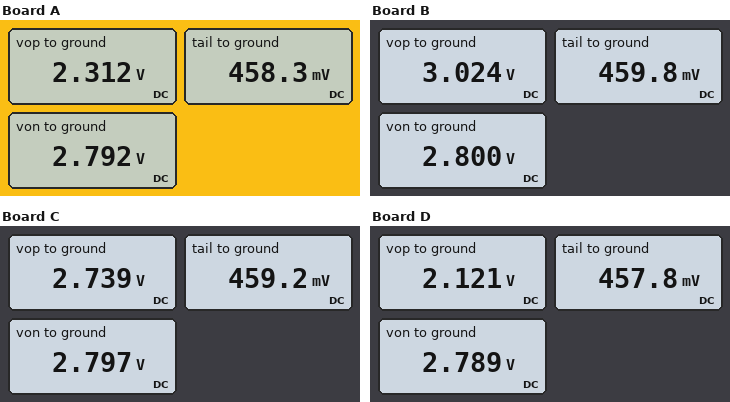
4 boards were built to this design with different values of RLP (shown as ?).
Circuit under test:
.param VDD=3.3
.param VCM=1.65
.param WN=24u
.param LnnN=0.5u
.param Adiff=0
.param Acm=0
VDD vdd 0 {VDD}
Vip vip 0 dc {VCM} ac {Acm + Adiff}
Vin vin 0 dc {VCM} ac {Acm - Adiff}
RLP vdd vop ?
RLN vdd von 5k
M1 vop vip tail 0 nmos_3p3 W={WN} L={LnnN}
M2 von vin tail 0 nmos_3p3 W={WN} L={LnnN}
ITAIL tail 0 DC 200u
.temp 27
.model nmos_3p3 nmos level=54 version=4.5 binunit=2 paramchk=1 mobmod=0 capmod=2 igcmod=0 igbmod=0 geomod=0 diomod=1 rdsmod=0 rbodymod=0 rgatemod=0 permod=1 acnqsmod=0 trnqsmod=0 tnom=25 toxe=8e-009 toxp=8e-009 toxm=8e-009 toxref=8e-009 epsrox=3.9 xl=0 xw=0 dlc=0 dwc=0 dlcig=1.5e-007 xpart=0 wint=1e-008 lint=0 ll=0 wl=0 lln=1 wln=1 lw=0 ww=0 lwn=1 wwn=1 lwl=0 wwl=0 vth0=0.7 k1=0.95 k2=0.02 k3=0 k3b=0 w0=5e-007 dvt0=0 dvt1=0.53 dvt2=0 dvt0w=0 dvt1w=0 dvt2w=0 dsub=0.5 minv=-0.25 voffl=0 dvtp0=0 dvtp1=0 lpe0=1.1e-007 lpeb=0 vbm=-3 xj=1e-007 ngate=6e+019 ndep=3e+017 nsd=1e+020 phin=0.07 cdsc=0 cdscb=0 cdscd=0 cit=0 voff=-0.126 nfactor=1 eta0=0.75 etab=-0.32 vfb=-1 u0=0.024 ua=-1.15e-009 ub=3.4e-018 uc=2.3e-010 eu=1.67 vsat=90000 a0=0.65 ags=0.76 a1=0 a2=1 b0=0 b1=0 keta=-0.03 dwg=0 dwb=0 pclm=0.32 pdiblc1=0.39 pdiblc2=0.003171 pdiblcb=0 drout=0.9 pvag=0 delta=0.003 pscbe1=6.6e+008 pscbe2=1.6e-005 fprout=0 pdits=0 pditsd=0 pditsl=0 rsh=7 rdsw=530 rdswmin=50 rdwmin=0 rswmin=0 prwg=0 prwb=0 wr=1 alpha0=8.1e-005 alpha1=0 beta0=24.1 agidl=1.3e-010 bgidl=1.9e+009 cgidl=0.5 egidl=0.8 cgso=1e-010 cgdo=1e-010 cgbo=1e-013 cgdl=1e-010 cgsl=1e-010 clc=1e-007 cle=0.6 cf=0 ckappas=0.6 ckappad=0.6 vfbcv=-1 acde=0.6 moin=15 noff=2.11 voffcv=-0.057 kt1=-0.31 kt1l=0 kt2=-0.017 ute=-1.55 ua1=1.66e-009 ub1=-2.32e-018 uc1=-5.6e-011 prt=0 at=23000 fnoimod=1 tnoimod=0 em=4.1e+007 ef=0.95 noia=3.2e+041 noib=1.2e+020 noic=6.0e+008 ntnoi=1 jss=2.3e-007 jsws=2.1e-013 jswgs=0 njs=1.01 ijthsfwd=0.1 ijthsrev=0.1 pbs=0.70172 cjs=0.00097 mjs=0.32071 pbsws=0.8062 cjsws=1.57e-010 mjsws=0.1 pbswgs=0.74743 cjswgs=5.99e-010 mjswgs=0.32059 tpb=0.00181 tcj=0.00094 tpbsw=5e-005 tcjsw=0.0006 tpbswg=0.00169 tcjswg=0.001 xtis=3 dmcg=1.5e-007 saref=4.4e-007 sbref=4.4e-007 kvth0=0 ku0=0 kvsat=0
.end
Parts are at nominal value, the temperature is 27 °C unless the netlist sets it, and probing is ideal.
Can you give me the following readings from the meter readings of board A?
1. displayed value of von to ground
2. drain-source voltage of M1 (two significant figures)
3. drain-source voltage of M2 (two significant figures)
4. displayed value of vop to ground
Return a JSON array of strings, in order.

["2.792 V", "1.9 V", "2.3 V", "2.312 V"]
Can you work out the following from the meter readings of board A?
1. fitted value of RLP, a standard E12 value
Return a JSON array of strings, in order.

["10 kΩ"]
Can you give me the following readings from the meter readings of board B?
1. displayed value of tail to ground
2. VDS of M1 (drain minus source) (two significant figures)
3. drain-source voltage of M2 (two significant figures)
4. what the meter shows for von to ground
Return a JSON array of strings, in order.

["459.8 mV", "2.6 V", "2.3 V", "2.800 V"]
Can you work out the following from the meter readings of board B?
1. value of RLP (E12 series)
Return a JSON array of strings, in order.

["2.7 kΩ"]
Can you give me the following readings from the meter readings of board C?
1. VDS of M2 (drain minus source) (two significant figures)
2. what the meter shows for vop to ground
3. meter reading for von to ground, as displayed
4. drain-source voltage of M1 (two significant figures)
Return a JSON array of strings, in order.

["2.3 V", "2.739 V", "2.797 V", "2.3 V"]
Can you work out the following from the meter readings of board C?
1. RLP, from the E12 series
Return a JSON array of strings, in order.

["5.6 kΩ"]
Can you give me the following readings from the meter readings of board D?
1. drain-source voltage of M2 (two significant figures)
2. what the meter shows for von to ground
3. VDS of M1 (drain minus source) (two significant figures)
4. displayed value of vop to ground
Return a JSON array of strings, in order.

["2.3 V", "2.789 V", "1.7 V", "2.121 V"]
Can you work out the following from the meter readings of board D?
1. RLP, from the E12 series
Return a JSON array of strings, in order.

["12 kΩ"]
